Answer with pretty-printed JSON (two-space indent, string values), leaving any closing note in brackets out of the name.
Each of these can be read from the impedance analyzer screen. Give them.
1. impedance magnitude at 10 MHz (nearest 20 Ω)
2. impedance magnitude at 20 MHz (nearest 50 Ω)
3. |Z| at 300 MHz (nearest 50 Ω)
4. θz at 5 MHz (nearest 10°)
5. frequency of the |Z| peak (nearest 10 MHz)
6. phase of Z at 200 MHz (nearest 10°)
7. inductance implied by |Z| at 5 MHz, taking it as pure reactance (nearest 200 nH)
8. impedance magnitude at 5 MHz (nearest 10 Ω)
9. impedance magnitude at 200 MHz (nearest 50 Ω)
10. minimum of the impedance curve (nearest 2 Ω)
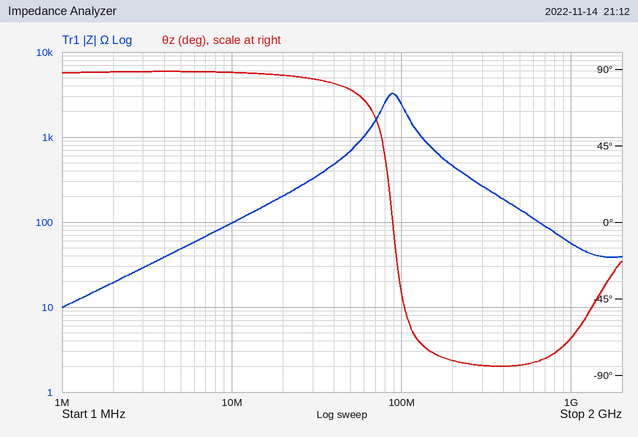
{
  "impedance magnitude at 10 MHz": "100 Ω",
  "impedance magnitude at 20 MHz": "200 Ω",
  "|Z| at 300 MHz": "250 Ω",
  "θz at 5 MHz": "90°",
  "frequency of the |Z| peak": "90 MHz",
  "phase of Z at 200 MHz": "-80°",
  "inductance implied by |Z| at 5 MHz, taking it as pure reactance": "1.6 µH",
  "impedance magnitude at 5 MHz": "50 Ω",
  "impedance magnitude at 200 MHz": "450 Ω",
  "minimum of the impedance curve": "10 Ω"
}
